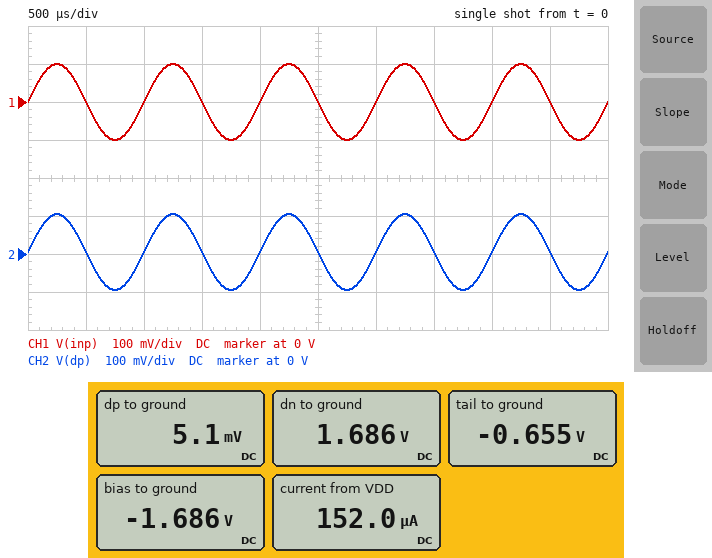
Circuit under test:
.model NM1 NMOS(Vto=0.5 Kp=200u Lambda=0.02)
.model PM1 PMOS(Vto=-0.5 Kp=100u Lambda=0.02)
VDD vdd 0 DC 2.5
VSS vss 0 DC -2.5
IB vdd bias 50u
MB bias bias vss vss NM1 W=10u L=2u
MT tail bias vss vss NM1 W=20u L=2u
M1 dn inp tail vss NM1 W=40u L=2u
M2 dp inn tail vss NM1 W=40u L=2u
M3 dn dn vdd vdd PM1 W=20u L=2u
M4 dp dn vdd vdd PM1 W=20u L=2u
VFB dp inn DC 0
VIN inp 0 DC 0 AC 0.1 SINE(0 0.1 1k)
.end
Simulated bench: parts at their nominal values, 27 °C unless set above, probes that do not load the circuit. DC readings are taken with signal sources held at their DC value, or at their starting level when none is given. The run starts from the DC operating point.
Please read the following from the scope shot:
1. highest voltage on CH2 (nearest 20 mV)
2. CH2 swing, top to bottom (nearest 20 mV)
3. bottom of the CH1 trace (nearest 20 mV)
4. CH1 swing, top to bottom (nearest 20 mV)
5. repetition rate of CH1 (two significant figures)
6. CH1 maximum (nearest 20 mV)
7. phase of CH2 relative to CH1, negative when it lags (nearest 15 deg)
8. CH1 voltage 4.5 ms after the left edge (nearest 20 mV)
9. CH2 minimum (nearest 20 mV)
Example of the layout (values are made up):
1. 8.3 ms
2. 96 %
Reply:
1. 100 mV
2. 200 mV
3. -100 mV
4. 200 mV
5. 1.0 kHz
6. 100 mV
7. 0 deg
8. 0 V
9. -100 mV
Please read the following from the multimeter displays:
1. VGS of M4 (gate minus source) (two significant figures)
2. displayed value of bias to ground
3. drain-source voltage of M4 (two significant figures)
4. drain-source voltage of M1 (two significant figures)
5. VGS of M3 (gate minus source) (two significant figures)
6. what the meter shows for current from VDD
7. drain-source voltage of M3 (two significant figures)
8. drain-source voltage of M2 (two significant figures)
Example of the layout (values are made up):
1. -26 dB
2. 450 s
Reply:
1. -810 mV
2. -1.686 V
3. -2.5 V
4. 2.3 V
5. -810 mV
6. 152.0 µA
7. -810 mV
8. 660 mV
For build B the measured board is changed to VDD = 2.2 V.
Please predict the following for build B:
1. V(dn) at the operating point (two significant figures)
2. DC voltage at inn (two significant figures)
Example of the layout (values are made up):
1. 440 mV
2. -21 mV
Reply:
1. 1.4 V
2. 4.2 mV
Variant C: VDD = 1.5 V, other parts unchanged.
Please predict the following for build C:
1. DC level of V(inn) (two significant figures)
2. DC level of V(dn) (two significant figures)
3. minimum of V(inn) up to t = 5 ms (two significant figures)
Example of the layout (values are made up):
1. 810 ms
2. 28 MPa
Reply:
1. 2.1 mV
2. 680 mV
3. -98 mV
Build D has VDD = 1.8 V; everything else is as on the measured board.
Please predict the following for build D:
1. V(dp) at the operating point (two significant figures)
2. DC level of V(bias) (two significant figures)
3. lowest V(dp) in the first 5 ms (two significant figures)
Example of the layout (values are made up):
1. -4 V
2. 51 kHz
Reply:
1. 3.0 mV
2. -1.7 V
3. -97 mV
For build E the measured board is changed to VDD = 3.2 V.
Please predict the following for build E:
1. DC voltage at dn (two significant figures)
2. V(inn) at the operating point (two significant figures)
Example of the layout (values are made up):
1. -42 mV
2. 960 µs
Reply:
1. 2.4 V
2. 7.2 mV
